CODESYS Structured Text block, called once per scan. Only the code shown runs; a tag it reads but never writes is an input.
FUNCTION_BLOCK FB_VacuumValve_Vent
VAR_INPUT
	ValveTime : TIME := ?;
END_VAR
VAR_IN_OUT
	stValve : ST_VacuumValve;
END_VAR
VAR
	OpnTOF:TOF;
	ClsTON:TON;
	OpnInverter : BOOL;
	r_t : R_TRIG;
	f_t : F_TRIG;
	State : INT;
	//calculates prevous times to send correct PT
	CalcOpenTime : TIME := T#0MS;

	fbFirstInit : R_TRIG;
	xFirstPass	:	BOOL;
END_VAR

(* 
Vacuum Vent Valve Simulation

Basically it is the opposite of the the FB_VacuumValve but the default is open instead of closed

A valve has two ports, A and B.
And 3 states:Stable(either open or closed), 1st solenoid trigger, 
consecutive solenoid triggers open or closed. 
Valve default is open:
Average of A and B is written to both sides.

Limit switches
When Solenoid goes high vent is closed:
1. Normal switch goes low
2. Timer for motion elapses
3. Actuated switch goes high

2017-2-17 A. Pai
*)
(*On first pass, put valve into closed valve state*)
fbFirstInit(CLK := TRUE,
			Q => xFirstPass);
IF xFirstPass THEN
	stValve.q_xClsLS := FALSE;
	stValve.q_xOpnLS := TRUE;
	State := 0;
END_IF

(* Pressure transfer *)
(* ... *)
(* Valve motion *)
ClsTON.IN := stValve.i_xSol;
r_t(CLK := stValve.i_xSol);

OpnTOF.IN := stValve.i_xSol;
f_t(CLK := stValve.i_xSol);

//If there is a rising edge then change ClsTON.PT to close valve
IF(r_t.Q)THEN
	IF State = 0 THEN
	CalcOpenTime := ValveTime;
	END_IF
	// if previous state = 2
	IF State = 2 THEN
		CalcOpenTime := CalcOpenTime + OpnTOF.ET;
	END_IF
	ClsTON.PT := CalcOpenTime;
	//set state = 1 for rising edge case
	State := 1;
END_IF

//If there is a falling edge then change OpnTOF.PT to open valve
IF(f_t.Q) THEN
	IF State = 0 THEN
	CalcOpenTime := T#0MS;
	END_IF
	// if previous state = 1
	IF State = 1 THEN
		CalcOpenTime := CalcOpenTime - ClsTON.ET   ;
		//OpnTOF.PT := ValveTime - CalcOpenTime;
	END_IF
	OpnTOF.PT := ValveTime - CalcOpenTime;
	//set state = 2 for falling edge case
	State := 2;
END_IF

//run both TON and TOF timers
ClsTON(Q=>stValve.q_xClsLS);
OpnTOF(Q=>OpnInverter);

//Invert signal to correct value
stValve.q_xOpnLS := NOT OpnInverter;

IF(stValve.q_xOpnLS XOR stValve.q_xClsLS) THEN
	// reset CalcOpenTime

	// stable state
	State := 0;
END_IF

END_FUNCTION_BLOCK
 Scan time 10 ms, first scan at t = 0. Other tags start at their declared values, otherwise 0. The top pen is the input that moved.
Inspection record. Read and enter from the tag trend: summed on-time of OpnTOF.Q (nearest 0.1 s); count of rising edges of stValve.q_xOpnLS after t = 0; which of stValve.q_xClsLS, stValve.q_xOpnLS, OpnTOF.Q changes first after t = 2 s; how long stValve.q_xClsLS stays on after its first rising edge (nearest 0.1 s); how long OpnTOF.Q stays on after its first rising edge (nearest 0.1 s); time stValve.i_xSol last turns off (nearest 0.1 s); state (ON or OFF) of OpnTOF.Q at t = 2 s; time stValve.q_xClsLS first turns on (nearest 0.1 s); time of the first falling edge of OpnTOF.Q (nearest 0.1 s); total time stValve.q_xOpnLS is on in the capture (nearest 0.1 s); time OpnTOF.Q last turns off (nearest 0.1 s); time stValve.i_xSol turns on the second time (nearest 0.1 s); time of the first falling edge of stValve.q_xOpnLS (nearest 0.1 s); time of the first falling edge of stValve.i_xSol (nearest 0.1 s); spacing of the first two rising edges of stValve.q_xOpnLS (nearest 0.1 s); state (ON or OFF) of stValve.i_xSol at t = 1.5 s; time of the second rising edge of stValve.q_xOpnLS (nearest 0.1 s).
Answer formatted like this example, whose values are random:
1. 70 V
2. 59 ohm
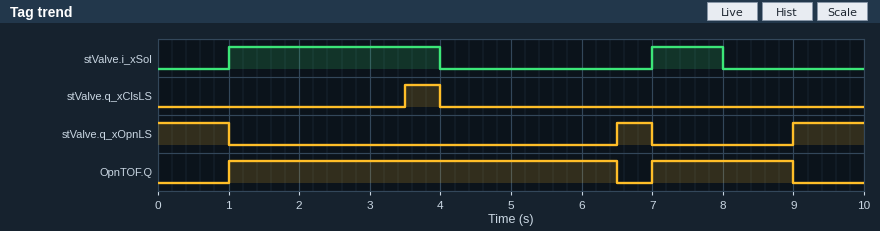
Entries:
1. 7.5 s
2. 2
3. stValve.q_xClsLS
4. 0.5 s
5. 5.5 s
6. 8.0 s
7. ON
8. 3.5 s
9. 6.5 s
10. 2.5 s
11. 9.0 s
12. 7.0 s
13. 1.0 s
14. 4.0 s
15. 2.5 s
16. ON
17. 9.0 s
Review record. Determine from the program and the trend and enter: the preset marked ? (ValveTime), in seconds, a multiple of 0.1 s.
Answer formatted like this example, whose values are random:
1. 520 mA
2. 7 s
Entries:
1. 2.5 s
